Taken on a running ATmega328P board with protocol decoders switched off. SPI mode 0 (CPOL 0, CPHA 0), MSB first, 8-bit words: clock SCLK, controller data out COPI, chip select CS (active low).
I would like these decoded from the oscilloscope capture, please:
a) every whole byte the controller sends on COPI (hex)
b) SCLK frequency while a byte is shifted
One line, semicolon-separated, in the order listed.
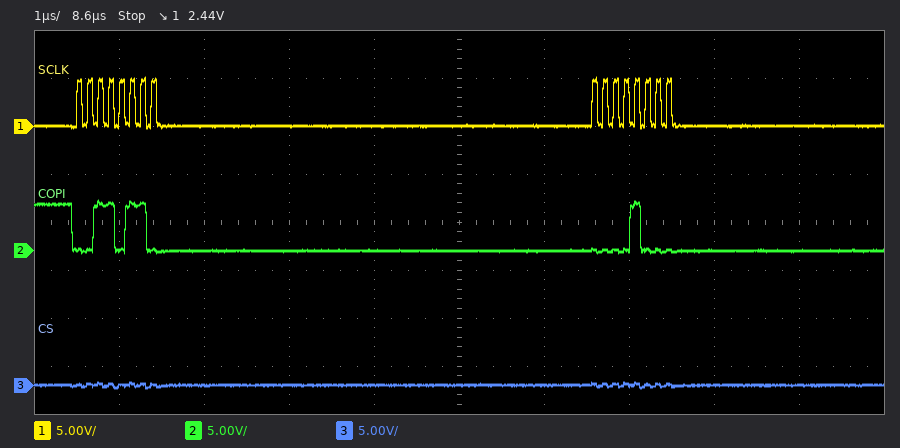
36 08; 8 MHz
